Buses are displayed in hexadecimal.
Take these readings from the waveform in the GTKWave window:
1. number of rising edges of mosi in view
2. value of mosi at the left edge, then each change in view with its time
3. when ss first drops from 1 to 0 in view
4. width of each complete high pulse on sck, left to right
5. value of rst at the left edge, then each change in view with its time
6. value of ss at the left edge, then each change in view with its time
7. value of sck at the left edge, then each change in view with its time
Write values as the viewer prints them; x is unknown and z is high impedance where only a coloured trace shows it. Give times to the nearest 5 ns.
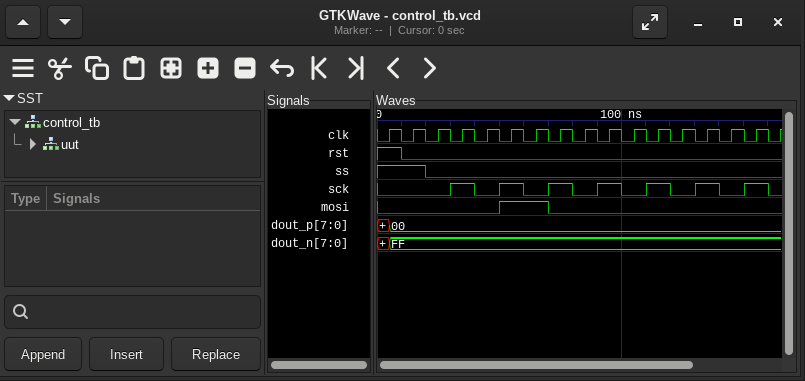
1
0, 1 at 50 ns, 0 at 70 ns
20 ns
10 ns, 10 ns, 10 ns, 10 ns, 10 ns, 10 ns, 10 ns
1, 0 at 10 ns
1, 0 at 20 ns
0, 1 at 30 ns, 0 at 40 ns, 1 at 50 ns, 0 at 60 ns, 1 at 70 ns, 0 at 80 ns, 1 at 90 ns, 0 at 100 ns, 1 at 110 ns, 0 at 120 ns, 1 at 130 ns, 0 at 140 ns, 1 at 150 ns, 0 at 160 ns
